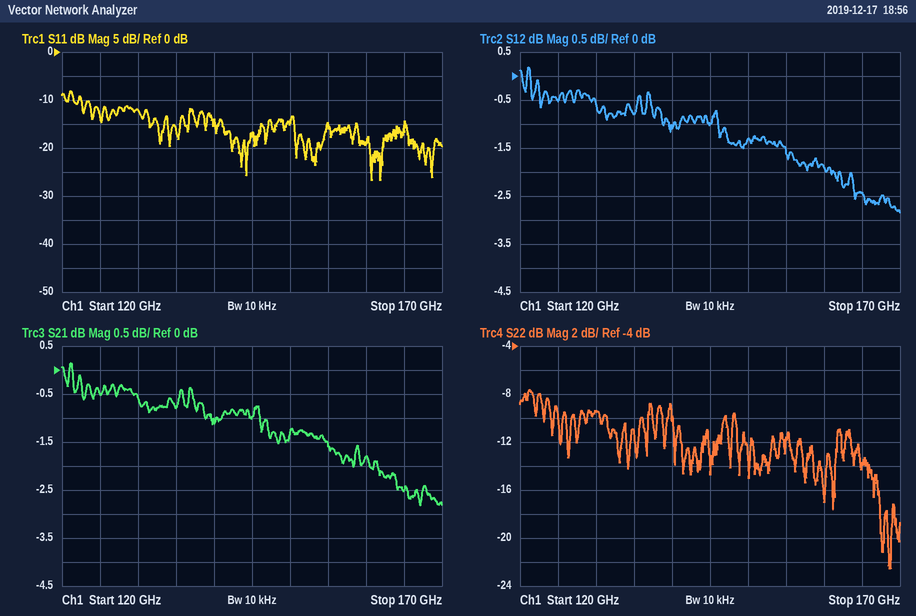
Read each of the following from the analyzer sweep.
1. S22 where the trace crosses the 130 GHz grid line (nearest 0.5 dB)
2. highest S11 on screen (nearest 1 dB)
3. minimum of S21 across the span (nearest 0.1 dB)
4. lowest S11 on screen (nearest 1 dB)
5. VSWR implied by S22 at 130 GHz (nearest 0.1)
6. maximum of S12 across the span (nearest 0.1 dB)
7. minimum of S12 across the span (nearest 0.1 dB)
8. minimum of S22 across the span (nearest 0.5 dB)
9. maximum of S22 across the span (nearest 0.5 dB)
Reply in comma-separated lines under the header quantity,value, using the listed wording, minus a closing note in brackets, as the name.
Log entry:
quantity,value
S22 where the trace crosses the 130 GHz grid line,-9.5 dB
highest S11 on screen,-8 dB
minimum of S21 across the span,-2.8 dB
lowest S11 on screen,-27 dB
VSWR implied by S22 at 130 GHz,2.0
maximum of S12 across the span,0.2 dB
minimum of S12 across the span,-2.8 dB
minimum of S22 across the span,-22.5 dB
maximum of S22 across the span,-7.5 dB
